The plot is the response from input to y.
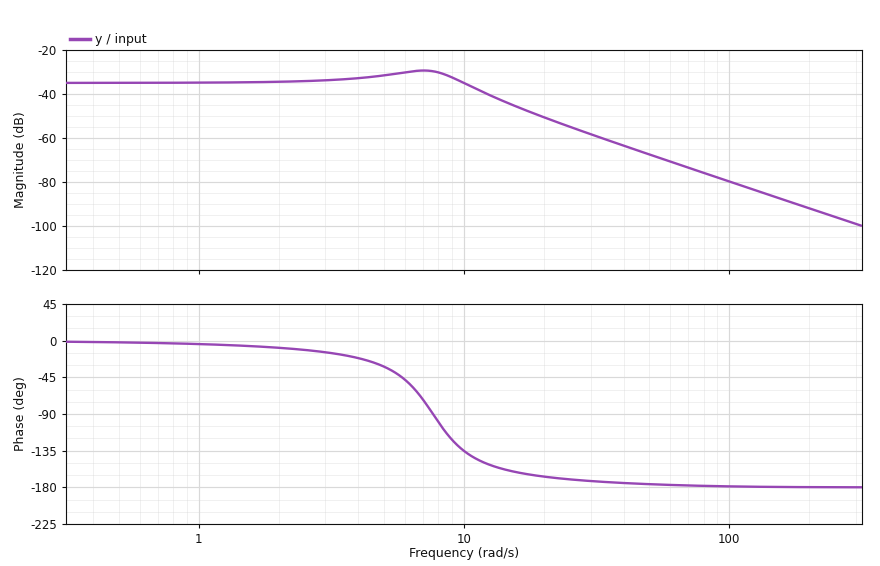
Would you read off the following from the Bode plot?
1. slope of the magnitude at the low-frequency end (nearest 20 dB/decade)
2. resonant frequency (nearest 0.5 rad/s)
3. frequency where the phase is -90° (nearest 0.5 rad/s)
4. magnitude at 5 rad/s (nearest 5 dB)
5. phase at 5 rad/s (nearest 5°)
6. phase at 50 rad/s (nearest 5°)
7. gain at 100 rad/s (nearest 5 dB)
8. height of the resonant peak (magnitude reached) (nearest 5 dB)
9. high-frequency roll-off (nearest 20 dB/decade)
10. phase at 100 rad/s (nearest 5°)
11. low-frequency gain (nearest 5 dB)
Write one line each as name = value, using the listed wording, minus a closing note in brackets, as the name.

slope of the magnitude at the low-frequency end = 0 dB/decade
resonant frequency = 7.0 rad/s
frequency where the phase is -90° = 7.5 rad/s
magnitude at 5 rad/s = -30 dB
phase at 5 rad/s = -30°
phase at 50 rad/s = -175°
gain at 100 rad/s = -80 dB
height of the resonant peak (magnitude reached) = -30 dB
high-frequency roll-off = -40 dB/decade
phase at 100 rad/s = -180°
low-frequency gain = -35 dB
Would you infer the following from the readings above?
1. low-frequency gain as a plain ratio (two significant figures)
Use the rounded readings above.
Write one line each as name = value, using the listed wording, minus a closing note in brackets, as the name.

low-frequency gain as a plain ratio = 0.018
